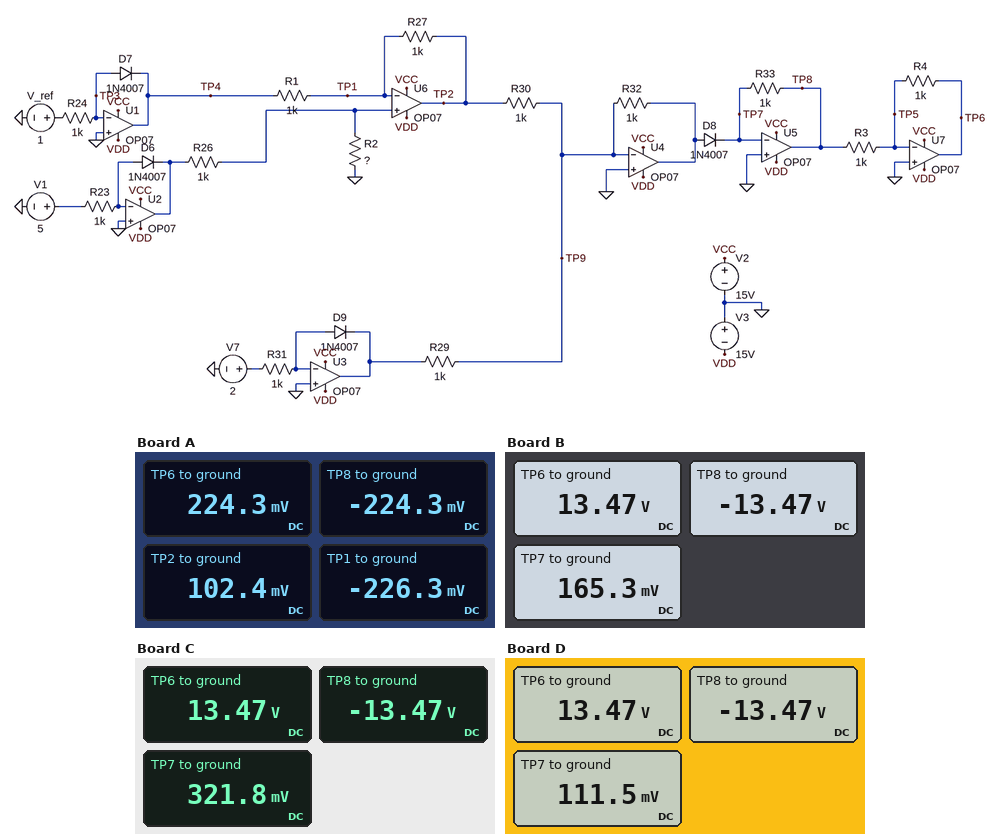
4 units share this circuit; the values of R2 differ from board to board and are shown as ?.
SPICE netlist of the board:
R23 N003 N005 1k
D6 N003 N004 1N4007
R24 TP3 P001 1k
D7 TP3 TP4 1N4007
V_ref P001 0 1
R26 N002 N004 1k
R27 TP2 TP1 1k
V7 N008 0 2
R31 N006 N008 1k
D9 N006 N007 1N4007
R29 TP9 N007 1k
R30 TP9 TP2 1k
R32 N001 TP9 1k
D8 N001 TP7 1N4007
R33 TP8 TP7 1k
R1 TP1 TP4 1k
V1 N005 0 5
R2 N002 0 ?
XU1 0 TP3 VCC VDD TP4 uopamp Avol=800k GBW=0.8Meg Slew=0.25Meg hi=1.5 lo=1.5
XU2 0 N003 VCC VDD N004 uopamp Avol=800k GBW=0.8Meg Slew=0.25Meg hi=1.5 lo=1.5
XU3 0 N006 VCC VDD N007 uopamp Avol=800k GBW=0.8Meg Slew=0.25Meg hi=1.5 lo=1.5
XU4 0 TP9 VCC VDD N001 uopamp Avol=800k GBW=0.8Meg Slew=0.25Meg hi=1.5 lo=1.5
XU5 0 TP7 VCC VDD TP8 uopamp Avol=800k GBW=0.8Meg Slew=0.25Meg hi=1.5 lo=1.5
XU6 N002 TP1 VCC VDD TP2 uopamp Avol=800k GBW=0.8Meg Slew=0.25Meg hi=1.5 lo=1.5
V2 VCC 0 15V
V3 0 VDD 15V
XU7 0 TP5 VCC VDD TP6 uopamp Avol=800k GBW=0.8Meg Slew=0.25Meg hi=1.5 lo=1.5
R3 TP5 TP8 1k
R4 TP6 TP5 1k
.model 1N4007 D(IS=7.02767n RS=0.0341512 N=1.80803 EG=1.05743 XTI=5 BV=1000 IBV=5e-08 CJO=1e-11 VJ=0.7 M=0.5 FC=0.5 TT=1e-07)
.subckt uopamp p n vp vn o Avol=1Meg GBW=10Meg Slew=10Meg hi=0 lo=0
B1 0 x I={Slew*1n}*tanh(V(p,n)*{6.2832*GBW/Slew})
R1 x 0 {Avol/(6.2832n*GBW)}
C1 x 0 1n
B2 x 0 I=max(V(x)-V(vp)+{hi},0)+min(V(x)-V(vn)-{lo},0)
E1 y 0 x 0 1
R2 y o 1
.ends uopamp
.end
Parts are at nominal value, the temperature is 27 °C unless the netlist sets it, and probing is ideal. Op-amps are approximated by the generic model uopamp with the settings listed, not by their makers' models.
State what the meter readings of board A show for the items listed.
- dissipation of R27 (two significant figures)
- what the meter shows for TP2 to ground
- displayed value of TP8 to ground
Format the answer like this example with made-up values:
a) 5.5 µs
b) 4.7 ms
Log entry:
a) 110 µW
b) 102.4 mV
c) -224.3 mV
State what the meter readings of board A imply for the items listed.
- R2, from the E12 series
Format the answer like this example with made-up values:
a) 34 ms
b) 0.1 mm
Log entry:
a) 560 Ω
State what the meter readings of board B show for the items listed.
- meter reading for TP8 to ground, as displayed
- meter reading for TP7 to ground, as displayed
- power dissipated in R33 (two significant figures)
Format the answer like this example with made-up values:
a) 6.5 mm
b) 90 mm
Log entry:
a) -13.47 V
b) 165.3 mV
c) 190 mW
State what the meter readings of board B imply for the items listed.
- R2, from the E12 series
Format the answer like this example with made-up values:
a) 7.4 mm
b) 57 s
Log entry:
a) 1.8 kΩ
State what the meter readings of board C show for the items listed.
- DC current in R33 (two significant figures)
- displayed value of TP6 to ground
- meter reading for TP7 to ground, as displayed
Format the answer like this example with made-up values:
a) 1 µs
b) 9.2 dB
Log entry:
a) 14 mA
b) 13.47 V
c) 321.8 mV
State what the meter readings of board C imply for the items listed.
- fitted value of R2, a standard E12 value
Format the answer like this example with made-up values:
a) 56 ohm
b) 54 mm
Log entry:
a) 3.3 kΩ
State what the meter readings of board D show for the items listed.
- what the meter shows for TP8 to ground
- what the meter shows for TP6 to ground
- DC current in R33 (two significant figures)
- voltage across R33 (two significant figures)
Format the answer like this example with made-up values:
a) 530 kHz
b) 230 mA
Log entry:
a) -13.47 V
b) 13.47 V
c) 14 mA
d) 14 V
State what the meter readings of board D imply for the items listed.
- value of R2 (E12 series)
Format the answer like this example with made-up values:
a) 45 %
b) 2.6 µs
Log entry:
a) 1.5 kΩ
